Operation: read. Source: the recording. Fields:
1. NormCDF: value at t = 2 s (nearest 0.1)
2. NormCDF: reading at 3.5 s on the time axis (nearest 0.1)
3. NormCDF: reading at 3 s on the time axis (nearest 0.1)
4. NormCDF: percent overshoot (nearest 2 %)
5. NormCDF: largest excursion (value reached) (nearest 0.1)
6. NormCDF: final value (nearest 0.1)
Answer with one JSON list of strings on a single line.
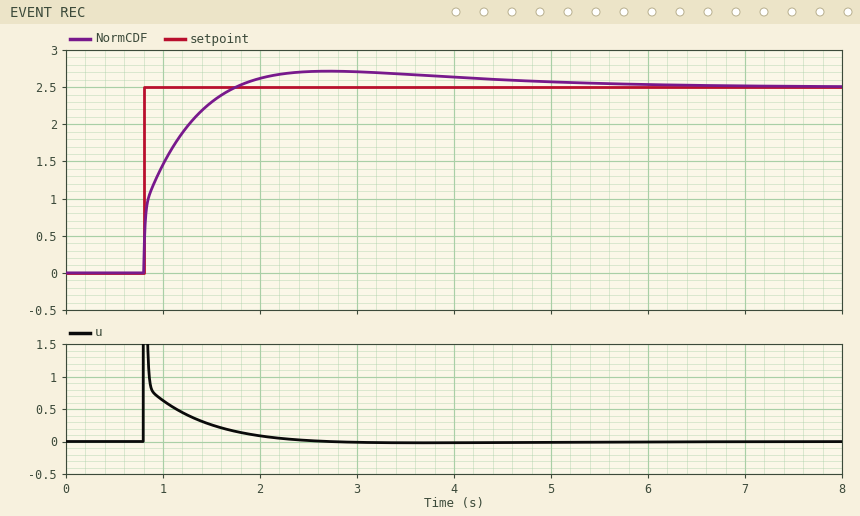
["2.6", "2.7", "2.7", "8 %", "2.7", "2.5"]
